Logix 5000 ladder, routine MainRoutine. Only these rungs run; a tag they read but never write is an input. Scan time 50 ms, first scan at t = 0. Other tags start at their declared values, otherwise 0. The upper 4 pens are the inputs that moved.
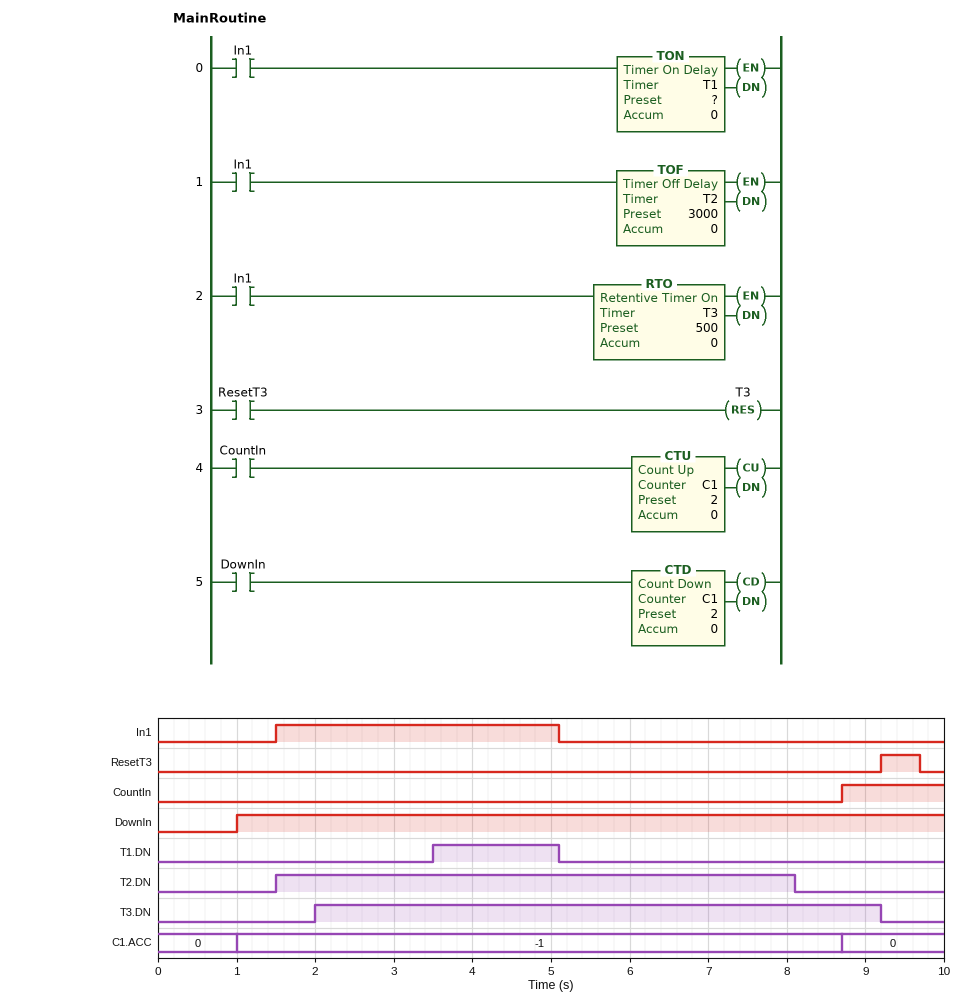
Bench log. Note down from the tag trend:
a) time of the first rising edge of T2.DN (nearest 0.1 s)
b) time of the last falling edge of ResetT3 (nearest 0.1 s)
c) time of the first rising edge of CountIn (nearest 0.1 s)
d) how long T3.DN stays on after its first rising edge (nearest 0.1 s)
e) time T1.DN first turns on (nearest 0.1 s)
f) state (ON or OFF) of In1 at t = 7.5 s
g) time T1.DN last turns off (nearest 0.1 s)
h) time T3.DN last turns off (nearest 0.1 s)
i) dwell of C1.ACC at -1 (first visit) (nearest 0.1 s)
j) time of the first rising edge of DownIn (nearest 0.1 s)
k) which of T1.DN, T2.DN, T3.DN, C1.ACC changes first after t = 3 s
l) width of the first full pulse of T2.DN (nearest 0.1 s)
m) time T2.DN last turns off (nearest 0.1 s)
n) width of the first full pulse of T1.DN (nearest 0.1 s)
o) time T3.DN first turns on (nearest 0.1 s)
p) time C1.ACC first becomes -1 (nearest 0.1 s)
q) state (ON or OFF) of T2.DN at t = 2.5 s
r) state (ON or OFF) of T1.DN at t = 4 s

1.5 s
9.7 s
8.7 s
7.2 s
3.5 s
OFF
5.1 s
9.2 s
7.7 s
1.0 s
T1.DN
6.6 s
8.1 s
1.6 s
2.0 s
1.0 s
ON
ON
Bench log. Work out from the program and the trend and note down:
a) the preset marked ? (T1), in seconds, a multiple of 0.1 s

2.0 s
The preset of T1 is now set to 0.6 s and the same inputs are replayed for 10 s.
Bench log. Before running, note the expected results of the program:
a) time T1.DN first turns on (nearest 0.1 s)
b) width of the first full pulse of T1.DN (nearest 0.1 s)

2.1 s
3.0 s
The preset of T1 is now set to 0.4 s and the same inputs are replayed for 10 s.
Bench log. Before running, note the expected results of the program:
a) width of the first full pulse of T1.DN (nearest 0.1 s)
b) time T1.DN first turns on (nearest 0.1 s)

3.2 s
1.9 s
